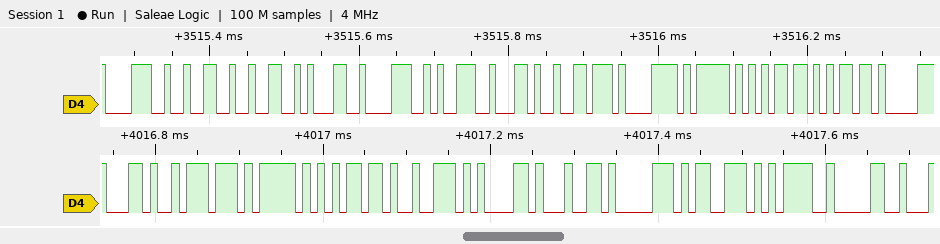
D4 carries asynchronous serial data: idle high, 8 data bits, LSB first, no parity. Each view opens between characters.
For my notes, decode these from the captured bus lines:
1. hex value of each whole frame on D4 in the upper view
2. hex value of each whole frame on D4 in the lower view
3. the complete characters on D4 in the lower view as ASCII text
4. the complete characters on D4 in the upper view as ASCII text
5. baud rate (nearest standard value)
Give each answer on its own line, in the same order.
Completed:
38, 32, 32, 31, 38, 39, 2C, 76, 78, 5F, 6D, 6D
2C, 77, 5F, 6D, 72, 61, 64, 70, 73, 3D, 30
",w_mradps=0"
"822189,vx_mm"
115200 baud
